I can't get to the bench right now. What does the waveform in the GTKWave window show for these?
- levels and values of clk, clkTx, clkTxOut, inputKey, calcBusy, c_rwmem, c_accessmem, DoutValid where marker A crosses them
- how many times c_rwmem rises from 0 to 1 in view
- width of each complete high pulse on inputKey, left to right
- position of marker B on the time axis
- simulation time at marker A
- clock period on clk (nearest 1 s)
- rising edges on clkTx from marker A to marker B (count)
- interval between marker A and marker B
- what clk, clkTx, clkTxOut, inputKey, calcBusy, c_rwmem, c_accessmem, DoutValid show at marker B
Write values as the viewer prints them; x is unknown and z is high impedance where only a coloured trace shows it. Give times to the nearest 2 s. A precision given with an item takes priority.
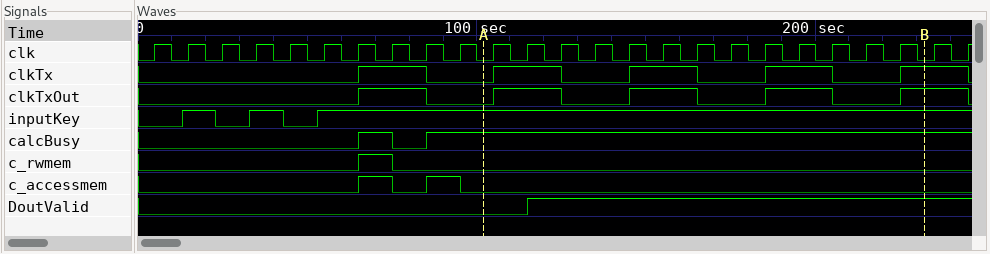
clk=0, clkTx=0, clkTxOut=0, inputKey=1, calcBusy=1, c_rwmem=0, c_accessmem=0, DoutValid=0
1
10 s, 10 s
232 s
102 s
10 s
4
130 s
clk=0, clkTx=1, clkTxOut=1, inputKey=1, calcBusy=1, c_rwmem=0, c_accessmem=0, DoutValid=1
